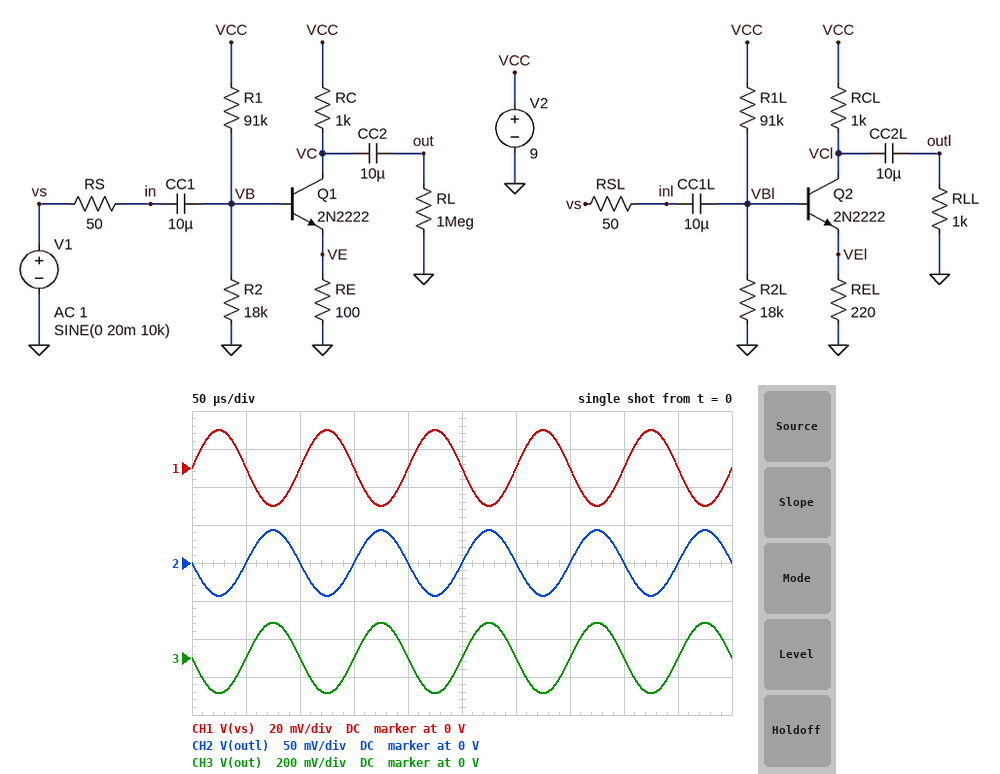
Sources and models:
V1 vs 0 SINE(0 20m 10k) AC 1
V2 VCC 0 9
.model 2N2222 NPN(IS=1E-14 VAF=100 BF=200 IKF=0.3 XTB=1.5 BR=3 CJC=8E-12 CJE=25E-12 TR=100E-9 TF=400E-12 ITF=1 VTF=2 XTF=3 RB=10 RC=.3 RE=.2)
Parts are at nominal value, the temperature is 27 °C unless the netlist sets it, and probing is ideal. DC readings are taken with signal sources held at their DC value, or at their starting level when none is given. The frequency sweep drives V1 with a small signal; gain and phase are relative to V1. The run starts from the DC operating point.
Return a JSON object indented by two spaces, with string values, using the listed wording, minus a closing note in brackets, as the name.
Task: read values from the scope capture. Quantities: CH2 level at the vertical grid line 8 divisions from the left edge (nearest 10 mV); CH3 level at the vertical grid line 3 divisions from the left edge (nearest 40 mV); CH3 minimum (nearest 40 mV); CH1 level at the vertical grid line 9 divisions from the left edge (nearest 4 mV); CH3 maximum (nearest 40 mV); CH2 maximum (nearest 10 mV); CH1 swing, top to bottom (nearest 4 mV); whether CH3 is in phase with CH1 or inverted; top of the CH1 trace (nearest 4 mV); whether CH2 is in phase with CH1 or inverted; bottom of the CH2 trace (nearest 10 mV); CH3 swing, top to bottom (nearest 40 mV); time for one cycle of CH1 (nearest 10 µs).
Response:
{
  "CH2 level at the vertical grid line 8 divisions from the left edge": "0 V",
  "CH3 level at the vertical grid line 3 divisions from the left edge": "0 V",
  "CH3 minimum": "-200 mV",
  "CH1 level at the vertical grid line 9 divisions from the left edge": "0 V",
  "CH3 maximum": "200 mV",
  "CH2 maximum": "40 mV",
  "CH1 swing, top to bottom": "40 mV",
  "whether CH3 is in phase with CH1 or inverted": "inverted",
  "top of the CH1 trace": "20 mV",
  "whether CH2 is in phase with CH1 or inverted": "inverted",
  "bottom of the CH2 trace": "-40 mV",
  "CH3 swing, top to bottom": "360 mV",
  "time for one cycle of CH1": "100 µs"
}
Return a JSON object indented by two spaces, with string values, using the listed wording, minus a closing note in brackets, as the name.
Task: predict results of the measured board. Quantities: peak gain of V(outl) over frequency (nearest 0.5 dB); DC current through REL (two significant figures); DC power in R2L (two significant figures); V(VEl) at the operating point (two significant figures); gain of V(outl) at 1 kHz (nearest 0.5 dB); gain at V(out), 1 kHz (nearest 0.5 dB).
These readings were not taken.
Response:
{
  "peak gain of V(outl) over frequency": "6.5 dB",
  "DC current through REL": "2.8 mA",
  "DC power in R2L": "92 µW",
  "V(VEl) at the operating point": "610 mV",
  "gain of V(outl) at 1 kHz": "6.5 dB",
  "gain at V(out), 1 kHz": "19.5 dB"
}
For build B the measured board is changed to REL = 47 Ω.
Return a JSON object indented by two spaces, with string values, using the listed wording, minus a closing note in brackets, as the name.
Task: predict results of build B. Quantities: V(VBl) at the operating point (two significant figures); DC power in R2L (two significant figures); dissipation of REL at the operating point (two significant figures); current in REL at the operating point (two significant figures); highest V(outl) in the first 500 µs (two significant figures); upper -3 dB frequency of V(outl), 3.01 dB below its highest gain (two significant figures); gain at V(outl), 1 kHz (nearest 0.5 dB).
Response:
{
  "V(VBl) at the operating point": "1.0 V",
  "DC power in R2L": "56 µW",
  "dissipation of REL at the operating point": "1.9 mW",
  "current in REL at the operating point": "6.4 mA",
  "highest V(outl) in the first 500 µs": "190 mV",
  "upper -3 dB frequency of V(outl), 3.01 dB below its highest gain": "23 MHz",
  "gain at V(outl), 1 kHz": "19.5 dB"
}
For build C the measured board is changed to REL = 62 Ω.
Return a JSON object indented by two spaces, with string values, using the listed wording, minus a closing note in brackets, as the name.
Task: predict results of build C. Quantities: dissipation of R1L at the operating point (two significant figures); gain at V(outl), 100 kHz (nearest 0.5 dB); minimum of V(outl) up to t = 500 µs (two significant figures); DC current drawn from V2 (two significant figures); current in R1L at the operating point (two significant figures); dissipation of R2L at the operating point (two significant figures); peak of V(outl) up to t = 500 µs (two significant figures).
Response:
{
  "dissipation of R1L at the operating point": "690 µW",
  "gain at V(outl), 100 kHz": "17.5 dB",
  "minimum of V(outl) up to t = 500 µs": "-150 mV",
  "DC current drawn from V2": "10 mA",
  "current in R1L at the operating point": "87 µA",
  "dissipation of R2L at the operating point": "62 µW",
  "peak of V(outl) up to t = 500 µs": "150 mV"
}
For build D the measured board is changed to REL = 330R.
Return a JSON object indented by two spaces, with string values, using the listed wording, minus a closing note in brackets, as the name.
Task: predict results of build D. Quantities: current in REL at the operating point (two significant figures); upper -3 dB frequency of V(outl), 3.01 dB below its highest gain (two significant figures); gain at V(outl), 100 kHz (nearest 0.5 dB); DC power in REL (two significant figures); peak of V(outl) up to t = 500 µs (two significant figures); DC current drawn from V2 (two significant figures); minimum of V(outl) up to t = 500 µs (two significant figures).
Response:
{
  "current in REL at the operating point": "2.0 mA",
  "upper -3 dB frequency of V(outl), 3.01 dB below its highest gain": "130 MHz",
  "gain at V(outl), 100 kHz": "3.0 dB",
  "DC power in REL": "1.4 mW",
  "peak of V(outl) up to t = 500 µs": "29 mV",
  "DC current drawn from V2": "6.7 mA",
  "minimum of V(outl) up to t = 500 µs": "-29 mV"
}
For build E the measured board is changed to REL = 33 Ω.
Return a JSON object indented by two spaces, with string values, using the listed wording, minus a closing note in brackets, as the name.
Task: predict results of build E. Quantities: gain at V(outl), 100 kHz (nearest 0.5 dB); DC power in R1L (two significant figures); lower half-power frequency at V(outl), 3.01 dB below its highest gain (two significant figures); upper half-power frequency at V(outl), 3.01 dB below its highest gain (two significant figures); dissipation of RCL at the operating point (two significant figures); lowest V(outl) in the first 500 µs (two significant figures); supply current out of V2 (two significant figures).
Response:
{
  "gain at V(outl), 100 kHz": "22.5 dB",
  "DC power in R1L": "710 µW",
  "lower half-power frequency at V(outl), 3.01 dB below its highest gain": "9.1 Hz",
  "upper half-power frequency at V(outl), 3.01 dB below its highest gain": "17 MHz",
  "dissipation of RCL at the operating point": "51 mW",
  "lowest V(outl) in the first 500 µs": "-270 mV",
  "supply current out of V2": "12 mA"
}
